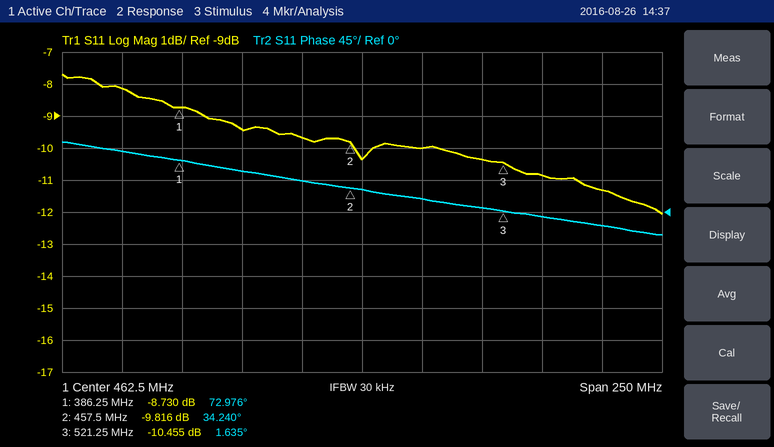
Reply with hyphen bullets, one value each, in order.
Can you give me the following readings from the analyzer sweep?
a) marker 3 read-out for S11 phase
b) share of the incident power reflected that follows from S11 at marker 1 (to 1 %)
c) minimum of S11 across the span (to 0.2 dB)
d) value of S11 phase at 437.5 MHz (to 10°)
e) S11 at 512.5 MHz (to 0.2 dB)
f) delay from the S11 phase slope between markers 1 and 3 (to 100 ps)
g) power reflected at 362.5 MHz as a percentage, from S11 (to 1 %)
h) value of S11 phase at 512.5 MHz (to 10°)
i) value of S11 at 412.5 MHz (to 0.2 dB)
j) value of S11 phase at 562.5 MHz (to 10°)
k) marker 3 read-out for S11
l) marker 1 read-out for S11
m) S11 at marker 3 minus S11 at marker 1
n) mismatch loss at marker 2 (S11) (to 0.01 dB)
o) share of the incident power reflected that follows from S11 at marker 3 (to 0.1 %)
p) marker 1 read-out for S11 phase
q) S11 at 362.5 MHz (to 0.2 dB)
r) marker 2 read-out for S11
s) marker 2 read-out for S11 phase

- 1.635°
- 13 %
- -12.0 dB
- 40°
- -10.4 dB
- 1.5 ns
- 15 %
- 10°
- -9.4 dB
- -20°
- -10.455 dB
- -8.730 dB
- -1.725 dB
- 0.48 dB
- 9.0 %
- 72.976°
- -8.2 dB
- -9.816 dB
- 34.240°
